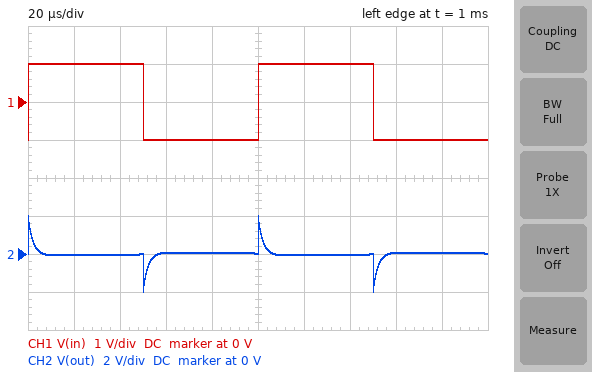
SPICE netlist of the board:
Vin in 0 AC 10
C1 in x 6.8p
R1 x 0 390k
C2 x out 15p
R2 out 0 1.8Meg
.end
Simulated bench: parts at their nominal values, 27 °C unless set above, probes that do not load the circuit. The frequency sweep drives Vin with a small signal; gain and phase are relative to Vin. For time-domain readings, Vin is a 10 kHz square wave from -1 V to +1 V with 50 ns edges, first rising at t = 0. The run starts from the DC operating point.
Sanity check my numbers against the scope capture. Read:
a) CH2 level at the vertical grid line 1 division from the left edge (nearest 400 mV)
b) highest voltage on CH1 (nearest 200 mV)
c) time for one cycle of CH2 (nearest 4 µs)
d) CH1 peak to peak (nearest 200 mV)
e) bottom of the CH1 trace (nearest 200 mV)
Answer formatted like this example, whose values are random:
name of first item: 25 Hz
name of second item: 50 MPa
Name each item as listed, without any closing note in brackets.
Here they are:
CH2 level at the vertical grid line 1 division from the left edge: 0 V
highest voltage on CH1: 1.0 V
time for one cycle of CH2: 100 µs
CH1 peak to peak: 2.0 V
bottom of the CH1 trace: -1.0 V
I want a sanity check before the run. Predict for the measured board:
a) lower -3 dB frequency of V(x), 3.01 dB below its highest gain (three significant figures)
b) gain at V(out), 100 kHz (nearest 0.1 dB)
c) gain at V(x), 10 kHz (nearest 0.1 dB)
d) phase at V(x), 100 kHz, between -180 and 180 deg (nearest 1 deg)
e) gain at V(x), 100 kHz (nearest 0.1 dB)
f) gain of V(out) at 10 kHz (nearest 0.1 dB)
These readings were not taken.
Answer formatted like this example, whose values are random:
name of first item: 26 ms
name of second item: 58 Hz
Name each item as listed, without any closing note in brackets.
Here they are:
lower -3 dB frequency of V(x), 3.01 dB below its highest gain: 74.0 kHz
gain at V(out), 100 kHz: -1.9 dB
gain at V(x), 10 kHz: -17.1 dB
phase at V(x), 100 kHz, between -180 and 180 deg: 36 deg
gain at V(x), 100 kHz: -1.9 dB
gain of V(out) at 10 kHz: -18.4 dB
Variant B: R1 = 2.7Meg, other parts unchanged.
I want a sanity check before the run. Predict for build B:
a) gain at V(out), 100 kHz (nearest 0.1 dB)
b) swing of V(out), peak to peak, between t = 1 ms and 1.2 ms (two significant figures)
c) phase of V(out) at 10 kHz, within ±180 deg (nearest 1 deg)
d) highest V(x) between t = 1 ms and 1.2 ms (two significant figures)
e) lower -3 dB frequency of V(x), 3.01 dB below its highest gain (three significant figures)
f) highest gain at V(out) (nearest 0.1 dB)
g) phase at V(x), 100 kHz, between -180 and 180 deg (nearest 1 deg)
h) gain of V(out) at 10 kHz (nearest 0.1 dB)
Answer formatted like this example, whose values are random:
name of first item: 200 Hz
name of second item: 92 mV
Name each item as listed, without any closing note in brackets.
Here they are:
gain at V(out), 100 kHz: -0.3 dB
swing of V(out), peak to peak, between t = 1 ms and 1.2 ms: 4.1 V
phase of V(out) at 10 kHz, within ±180 deg: 80 deg
highest V(x) between t = 1 ms and 1.2 ms: 1.9 V
lower -3 dB frequency of V(x), 3.01 dB below its highest gain: 24.3 kHz
highest gain at V(out): 0 dB
phase at V(x), 100 kHz, between -180 and 180 deg: 12 deg
gain of V(out) at 10 kHz: -8.9 dB
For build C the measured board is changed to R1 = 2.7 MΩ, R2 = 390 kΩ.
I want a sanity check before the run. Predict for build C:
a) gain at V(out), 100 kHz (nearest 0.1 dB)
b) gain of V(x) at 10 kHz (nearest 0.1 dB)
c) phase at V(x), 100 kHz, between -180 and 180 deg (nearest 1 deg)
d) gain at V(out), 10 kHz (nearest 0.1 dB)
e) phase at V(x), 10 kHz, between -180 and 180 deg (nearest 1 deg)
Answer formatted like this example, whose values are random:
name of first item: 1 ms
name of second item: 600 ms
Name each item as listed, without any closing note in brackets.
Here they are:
gain at V(out), 100 kHz: -2.7 dB
gain of V(x) at 10 kHz: -10.5 dB
phase at V(x), 100 kHz, between -180 and 180 deg: 29 deg
gain at V(out), 10 kHz: -19.7 dB
phase at V(x), 10 kHz, between -180 and 180 deg: 28 deg
